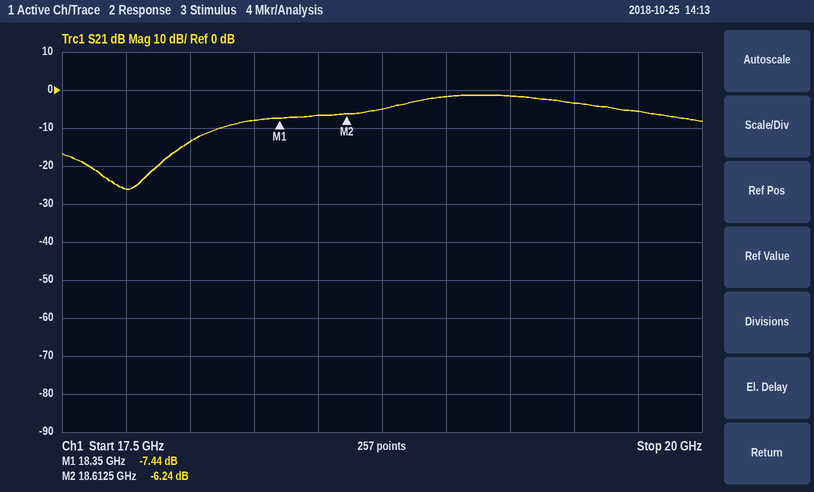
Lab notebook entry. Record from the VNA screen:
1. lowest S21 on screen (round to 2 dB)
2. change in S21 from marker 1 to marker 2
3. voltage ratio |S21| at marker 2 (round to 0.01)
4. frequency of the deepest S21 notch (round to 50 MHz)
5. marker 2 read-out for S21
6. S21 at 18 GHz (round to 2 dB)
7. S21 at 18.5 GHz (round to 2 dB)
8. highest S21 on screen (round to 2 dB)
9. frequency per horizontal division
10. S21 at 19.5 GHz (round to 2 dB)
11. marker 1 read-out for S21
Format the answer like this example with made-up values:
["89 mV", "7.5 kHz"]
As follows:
["-26 dB", "1.20 dB", "0.49", "17.75 GHz", "-6.24 dB", "-14 dB", "-6 dB", "-2 dB", "250 MHz", "-4 dB", "-7.44 dB"]
